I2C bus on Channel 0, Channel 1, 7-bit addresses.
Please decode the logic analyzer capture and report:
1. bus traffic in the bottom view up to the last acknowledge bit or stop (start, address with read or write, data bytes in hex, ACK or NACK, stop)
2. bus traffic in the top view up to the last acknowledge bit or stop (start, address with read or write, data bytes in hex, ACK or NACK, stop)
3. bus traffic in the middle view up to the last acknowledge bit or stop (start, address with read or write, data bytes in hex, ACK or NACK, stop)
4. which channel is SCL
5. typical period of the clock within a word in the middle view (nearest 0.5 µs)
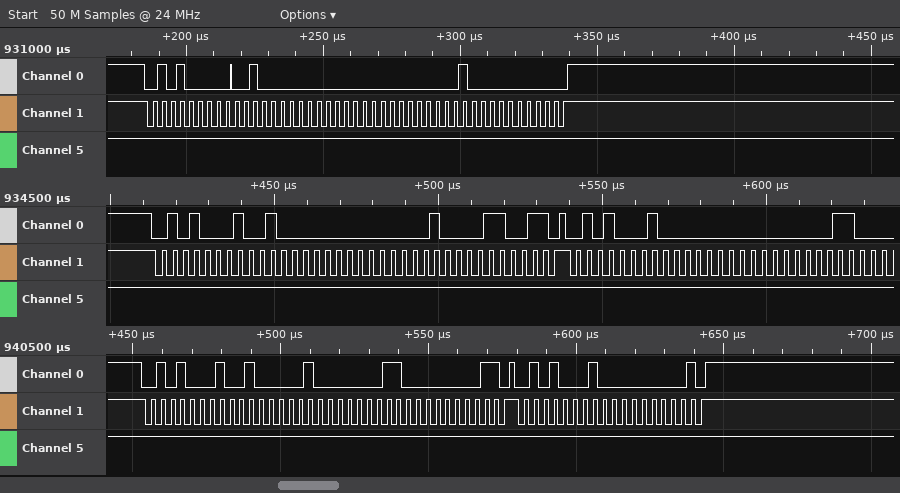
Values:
start, address 28 read ACK, 41 ACK, 03 ACK, 01 NACK, stop, start, address 28 read ACK, 00 NACK, stop
start, address 28 write ACK, 20 ACK, 00 ACK, 01 ACK, 00 ACK, stop
start, address 28 read ACK, 40 ACK, 01 ACK, 19 NACK, stop, start, address 28 read ACK, 00 ACK, 03 ACK
Channel 1
3.5 µs
